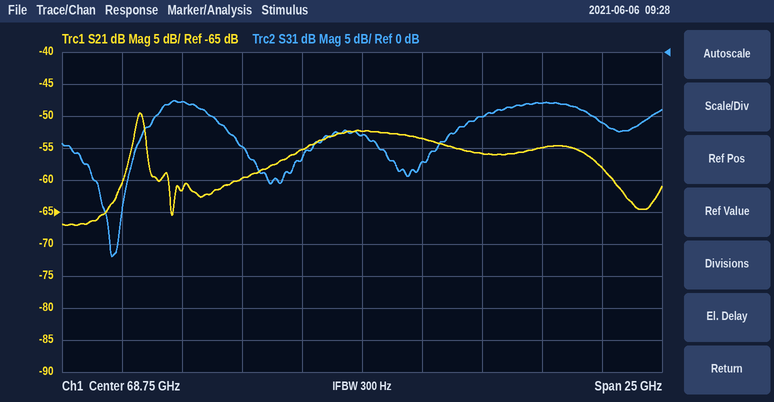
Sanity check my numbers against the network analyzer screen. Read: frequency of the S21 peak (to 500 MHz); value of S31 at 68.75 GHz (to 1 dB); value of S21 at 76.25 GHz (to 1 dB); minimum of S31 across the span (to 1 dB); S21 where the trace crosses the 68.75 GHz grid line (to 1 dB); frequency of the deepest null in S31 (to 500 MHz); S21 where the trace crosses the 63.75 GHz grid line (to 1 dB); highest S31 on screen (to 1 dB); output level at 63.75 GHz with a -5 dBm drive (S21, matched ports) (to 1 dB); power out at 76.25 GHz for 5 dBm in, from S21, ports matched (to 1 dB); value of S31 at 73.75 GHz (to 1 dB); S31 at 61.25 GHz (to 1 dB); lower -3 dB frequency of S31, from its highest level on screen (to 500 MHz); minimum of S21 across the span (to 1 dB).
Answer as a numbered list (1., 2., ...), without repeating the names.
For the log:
1. 59.5 GHz
2. -13 dB
3. -55 dB
4. -32 dB
5. -52 dB
6. 58.5 GHz
7. -60 dB
8. -8 dB
9. -65 dBm
10. -50 dBm
11. -10 dB
12. -8 dB
13. 60.0 GHz
14. -67 dB
